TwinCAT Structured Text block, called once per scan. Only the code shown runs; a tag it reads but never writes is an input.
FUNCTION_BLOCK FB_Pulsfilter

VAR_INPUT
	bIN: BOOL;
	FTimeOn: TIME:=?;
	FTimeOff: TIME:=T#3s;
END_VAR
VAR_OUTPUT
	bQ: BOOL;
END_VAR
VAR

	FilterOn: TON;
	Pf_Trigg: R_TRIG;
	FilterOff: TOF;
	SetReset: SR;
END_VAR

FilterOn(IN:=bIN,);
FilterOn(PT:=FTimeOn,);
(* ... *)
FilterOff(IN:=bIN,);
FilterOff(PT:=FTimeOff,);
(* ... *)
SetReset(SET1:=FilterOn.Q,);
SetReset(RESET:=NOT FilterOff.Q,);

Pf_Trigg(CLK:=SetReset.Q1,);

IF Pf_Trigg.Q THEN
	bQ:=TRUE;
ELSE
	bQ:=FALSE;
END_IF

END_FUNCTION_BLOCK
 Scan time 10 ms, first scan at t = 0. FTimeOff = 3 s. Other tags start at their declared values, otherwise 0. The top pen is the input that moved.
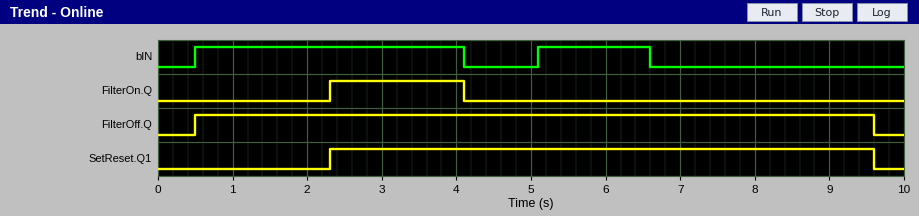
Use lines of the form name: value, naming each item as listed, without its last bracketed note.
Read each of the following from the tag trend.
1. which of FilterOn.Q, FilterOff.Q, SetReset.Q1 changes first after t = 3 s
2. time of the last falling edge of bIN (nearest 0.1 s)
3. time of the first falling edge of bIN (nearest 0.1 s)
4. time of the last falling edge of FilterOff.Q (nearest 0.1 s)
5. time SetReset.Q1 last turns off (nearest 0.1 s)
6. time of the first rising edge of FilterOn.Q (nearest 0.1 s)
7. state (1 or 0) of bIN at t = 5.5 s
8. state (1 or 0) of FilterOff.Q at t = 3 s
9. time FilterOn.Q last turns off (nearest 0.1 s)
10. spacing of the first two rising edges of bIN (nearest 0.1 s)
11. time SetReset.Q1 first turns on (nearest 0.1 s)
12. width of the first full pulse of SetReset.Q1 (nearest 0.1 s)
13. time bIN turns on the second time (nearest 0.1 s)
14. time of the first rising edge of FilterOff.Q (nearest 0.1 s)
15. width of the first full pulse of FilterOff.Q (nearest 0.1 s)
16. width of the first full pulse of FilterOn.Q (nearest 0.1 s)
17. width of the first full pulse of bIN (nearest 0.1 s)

which of FilterOn.Q, FilterOff.Q, SetReset.Q1 changes first after t = 3 s: FilterOn.Q
time of the last falling edge of bIN: 6.6 s
time of the first falling edge of bIN: 4.1 s
time of the last falling edge of FilterOff.Q: 9.6 s
time SetReset.Q1 last turns off: 9.6 s
time of the first rising edge of FilterOn.Q: 2.3 s
state (1 or 0) of bIN at t = 5.5 s: 1
state (1 or 0) of FilterOff.Q at t = 3 s: 1
time FilterOn.Q last turns off: 4.1 s
spacing of the first two rising edges of bIN: 4.6 s
time SetReset.Q1 first turns on: 2.3 s
width of the first full pulse of SetReset.Q1: 7.3 s
time bIN turns on the second time: 5.1 s
time of the first rising edge of FilterOff.Q: 0.5 s
width of the first full pulse of FilterOff.Q: 9.1 s
width of the first full pulse of FilterOn.Q: 1.8 s
width of the first full pulse of bIN: 3.6 s
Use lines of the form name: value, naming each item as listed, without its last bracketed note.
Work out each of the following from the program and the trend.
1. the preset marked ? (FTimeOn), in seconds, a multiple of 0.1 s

the preset marked ? (FTimeOn), in seconds, a multiple of 0.1 s: 1.8 s
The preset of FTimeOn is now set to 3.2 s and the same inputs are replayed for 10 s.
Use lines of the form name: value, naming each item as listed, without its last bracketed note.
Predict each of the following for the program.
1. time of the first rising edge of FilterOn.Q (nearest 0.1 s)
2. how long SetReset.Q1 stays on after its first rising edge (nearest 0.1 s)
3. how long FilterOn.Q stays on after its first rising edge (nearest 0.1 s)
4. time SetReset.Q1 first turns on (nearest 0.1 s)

time of the first rising edge of FilterOn.Q: 3.7 s
how long SetReset.Q1 stays on after its first rising edge: 5.9 s
how long FilterOn.Q stays on after its first rising edge: 0.4 s
time SetReset.Q1 first turns on: 3.7 s
